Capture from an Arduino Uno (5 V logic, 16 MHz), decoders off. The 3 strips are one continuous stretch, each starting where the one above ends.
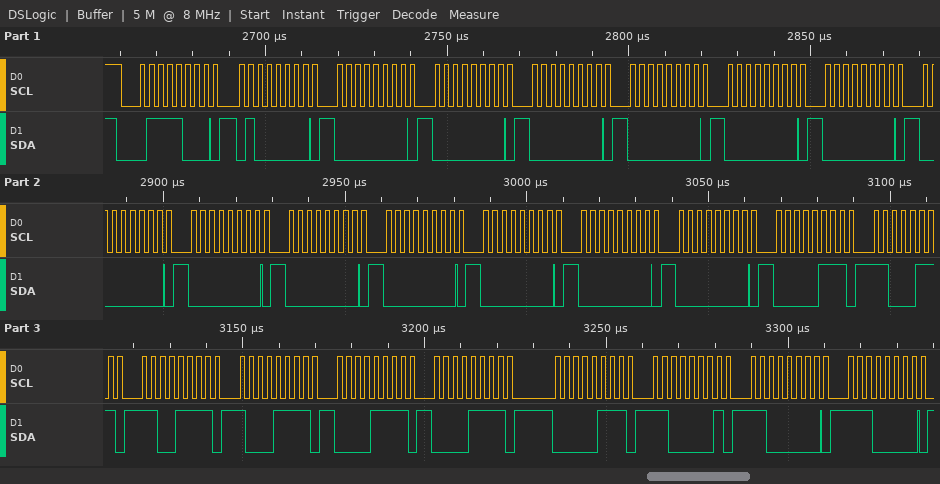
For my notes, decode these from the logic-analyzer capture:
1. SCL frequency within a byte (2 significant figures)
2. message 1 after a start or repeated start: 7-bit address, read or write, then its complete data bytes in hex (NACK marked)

400 kHz
0x3C write: 40 00 00 00 00 00 00 00 00 00 00 00 00 00 07 C7 CF 8F 0F 0F 07 C1 C0 E0
